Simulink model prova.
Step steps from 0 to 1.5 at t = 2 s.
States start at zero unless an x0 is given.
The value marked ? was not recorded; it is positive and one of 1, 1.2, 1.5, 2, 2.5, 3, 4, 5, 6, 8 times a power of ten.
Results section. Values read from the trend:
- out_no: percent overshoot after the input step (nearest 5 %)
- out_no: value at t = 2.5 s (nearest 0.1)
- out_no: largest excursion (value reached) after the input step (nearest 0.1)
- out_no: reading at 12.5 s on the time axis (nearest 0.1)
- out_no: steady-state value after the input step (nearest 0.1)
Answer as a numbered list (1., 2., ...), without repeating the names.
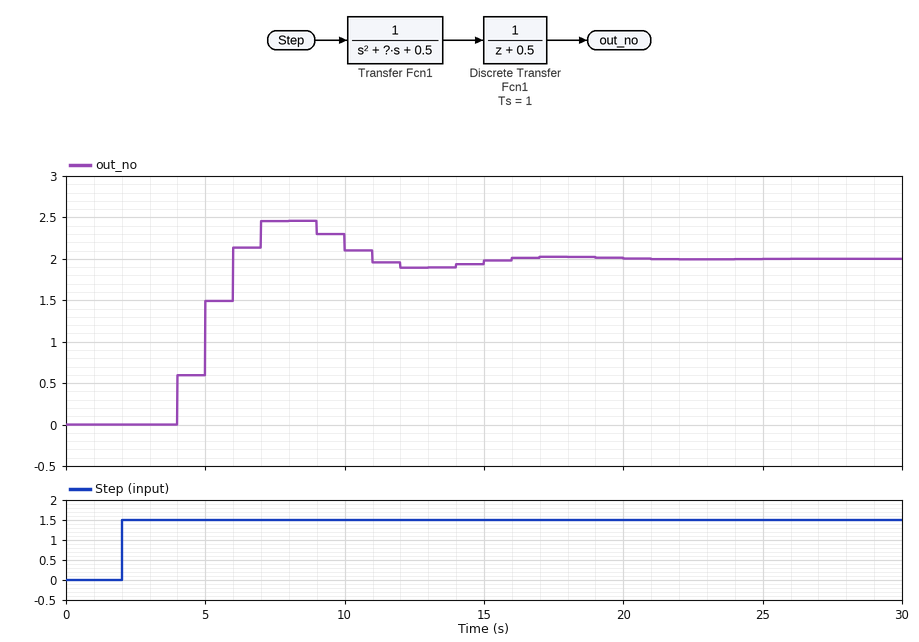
1. 25 %
2. 0.0
3. 2.5
4. 1.9
5. 2.0
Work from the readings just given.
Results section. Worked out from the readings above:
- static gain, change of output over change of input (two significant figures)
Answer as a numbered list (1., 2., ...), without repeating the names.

1. 1.3
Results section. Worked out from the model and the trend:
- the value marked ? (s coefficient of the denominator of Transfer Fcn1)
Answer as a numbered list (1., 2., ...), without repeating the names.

1. 0.6
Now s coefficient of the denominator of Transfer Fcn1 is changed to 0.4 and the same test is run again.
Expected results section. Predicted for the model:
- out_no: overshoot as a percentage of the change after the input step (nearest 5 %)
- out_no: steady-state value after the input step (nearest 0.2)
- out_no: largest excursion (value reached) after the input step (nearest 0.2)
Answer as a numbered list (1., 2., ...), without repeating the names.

1. 40 %
2. 2.0
3. 2.8
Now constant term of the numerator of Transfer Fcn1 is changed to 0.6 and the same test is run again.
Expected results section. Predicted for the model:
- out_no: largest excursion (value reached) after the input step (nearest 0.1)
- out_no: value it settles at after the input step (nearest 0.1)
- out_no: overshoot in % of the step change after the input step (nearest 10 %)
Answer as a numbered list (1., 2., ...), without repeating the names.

1. 1.5
2. 1.2
3. 20 %
